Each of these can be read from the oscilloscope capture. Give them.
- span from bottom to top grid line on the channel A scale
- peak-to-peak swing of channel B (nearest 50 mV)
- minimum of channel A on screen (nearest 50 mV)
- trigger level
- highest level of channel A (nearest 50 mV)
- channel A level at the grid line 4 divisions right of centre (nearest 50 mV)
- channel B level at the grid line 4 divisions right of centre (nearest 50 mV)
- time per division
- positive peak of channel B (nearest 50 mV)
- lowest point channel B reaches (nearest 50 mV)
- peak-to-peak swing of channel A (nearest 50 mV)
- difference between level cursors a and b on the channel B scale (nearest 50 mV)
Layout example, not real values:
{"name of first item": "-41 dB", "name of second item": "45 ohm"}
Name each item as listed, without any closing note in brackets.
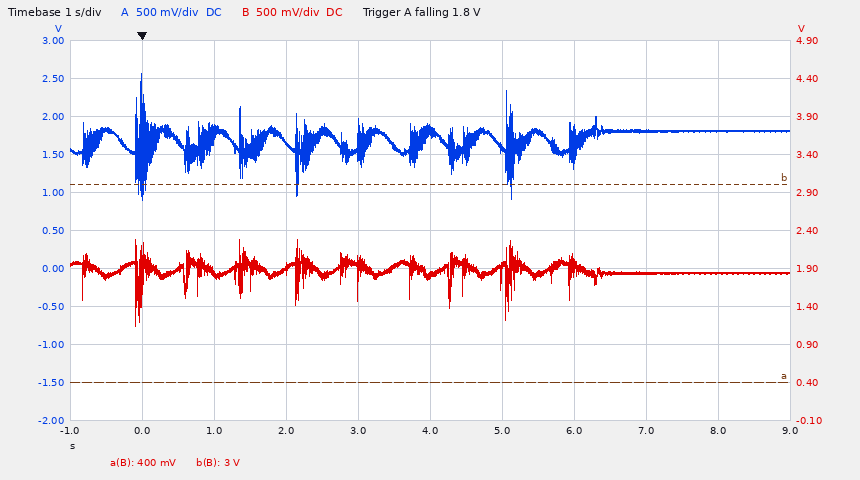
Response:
{"span from bottom to top grid line on the channel A scale": "5 V", "peak-to-peak swing of channel B": "1.15 V", "minimum of channel A on screen": "900 mV", "trigger level": "1.8 V", "highest level of channel A": "2.55 V", "channel A level at the grid line 4 divisions right of centre": "1.80 V", "channel B level at the grid line 4 divisions right of centre": "1.85 V", "time per division": "1 s", "positive peak of channel B": "2.30 V", "lowest point channel B reaches": "1.15 V", "peak-to-peak swing of channel A": "1.65 V", "difference between level cursors a and b on the channel B scale": "2.60 V"}
